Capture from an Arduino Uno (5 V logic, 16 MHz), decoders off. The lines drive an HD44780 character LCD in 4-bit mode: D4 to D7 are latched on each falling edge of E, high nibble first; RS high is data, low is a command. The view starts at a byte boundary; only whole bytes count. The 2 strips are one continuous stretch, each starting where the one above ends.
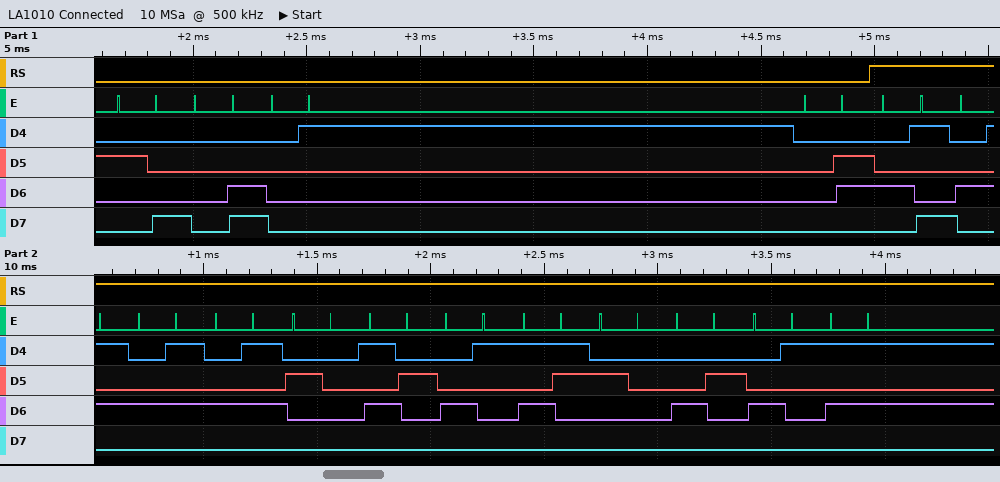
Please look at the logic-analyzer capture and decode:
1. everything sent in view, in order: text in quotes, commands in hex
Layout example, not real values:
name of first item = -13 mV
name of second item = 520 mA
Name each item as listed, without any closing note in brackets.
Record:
everything sent in view, in order: text in quotes, commands in hex = 0x28 0x0C 0x01 0x06 "IEEE RAS BAU"
